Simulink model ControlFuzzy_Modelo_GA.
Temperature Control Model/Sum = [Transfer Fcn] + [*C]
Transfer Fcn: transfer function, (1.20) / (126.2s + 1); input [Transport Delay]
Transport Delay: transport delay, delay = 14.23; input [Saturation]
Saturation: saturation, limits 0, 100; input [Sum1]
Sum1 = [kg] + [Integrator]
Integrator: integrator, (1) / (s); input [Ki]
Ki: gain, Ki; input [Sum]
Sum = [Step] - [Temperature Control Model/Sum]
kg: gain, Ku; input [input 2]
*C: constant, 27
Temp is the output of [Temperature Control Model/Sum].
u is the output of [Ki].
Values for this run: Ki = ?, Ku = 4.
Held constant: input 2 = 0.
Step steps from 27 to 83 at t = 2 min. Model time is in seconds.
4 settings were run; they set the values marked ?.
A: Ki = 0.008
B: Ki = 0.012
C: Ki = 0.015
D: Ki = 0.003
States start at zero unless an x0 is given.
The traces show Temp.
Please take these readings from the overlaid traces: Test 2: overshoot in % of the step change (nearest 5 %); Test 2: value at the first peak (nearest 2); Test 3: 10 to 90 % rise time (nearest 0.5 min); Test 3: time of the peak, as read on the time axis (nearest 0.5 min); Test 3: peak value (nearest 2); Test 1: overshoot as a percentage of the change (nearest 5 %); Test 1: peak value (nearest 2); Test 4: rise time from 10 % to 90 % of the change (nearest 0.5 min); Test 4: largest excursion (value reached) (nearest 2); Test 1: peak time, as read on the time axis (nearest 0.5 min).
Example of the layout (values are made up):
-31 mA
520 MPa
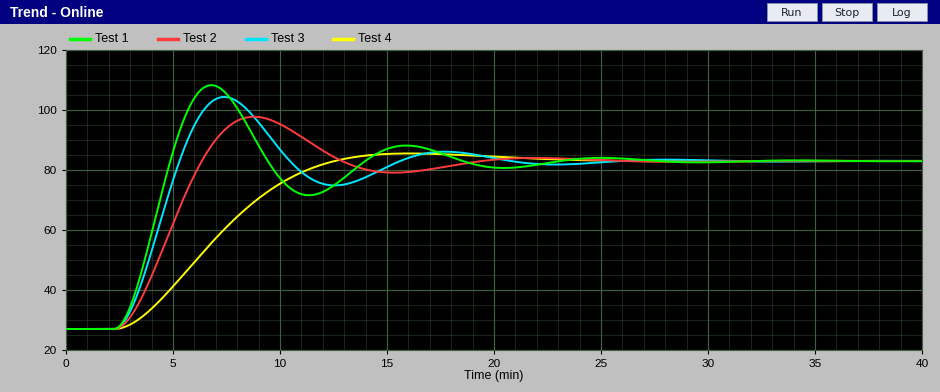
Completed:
25 %
98
2.0 min
7.5 min
104
45 %
108
6.5 min
86
7.0 min
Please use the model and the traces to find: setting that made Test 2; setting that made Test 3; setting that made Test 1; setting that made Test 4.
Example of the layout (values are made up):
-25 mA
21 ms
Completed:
A
B
C
D
